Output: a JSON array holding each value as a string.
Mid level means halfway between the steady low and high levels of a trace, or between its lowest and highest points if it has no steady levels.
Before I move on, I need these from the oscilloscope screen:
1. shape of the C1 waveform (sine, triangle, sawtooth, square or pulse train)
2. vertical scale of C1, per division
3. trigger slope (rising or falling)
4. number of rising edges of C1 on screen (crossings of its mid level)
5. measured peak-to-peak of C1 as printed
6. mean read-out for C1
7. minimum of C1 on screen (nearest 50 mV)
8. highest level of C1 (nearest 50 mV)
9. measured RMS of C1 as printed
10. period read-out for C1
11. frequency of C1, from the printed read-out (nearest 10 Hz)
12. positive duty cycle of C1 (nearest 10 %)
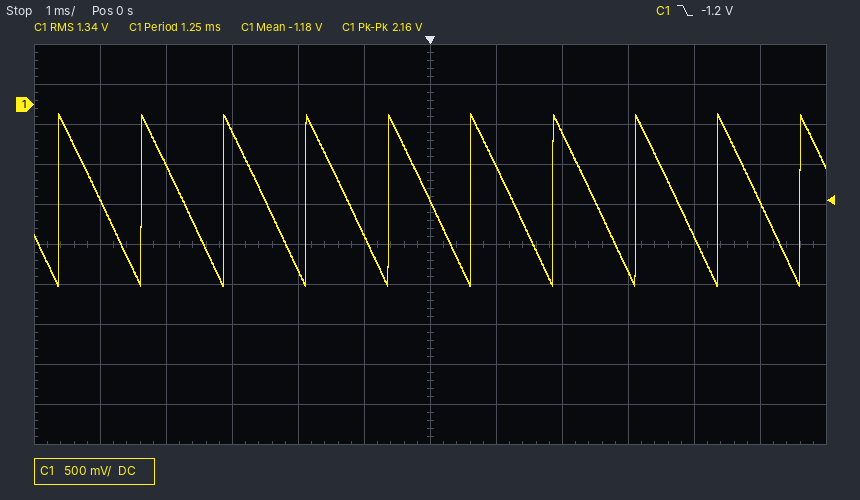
["sawtooth", "500 mV", "falling", "10", "2.16 V", "-1.18 V", "-2.25 V", "-100 mV", "1.34 V", "1.25 ms", "800 Hz", "50 %"]
